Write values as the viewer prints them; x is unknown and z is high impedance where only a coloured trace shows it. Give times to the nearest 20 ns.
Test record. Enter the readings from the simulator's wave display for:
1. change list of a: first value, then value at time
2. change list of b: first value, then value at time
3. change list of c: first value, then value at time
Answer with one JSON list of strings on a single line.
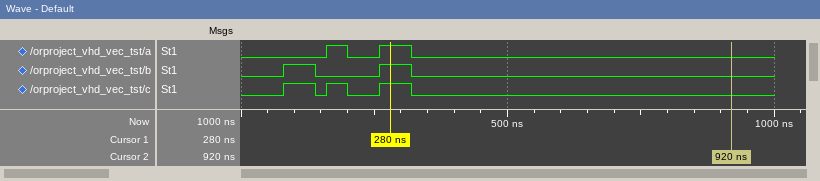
["0, 1 at 160 ns, 0 at 200 ns, 1 at 260 ns, 0 at 320 ns", "0, 1 at 80 ns, 0 at 140 ns, 1 at 260 ns, 0 at 320 ns", "0, 1 at 80 ns, 0 at 140 ns, 1 at 160 ns, 0 at 200 ns, 1 at 260 ns, 0 at 320 ns"]
